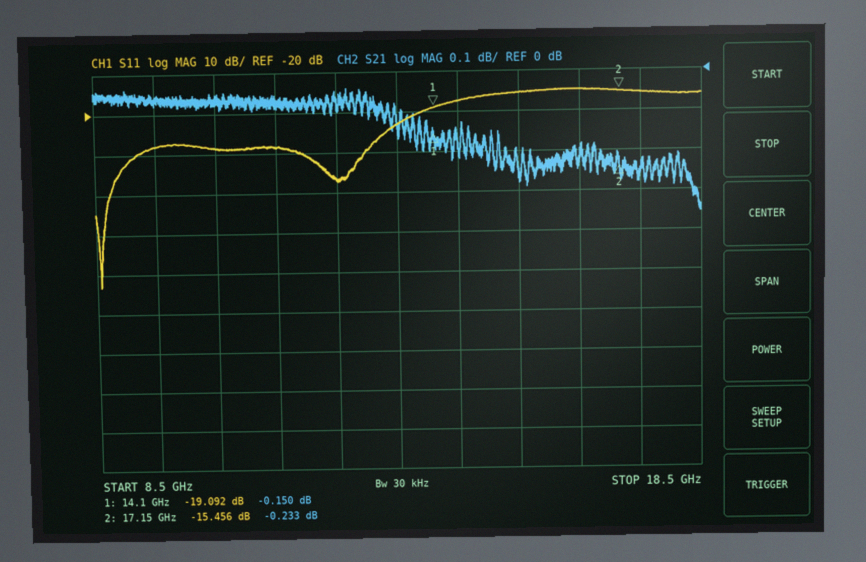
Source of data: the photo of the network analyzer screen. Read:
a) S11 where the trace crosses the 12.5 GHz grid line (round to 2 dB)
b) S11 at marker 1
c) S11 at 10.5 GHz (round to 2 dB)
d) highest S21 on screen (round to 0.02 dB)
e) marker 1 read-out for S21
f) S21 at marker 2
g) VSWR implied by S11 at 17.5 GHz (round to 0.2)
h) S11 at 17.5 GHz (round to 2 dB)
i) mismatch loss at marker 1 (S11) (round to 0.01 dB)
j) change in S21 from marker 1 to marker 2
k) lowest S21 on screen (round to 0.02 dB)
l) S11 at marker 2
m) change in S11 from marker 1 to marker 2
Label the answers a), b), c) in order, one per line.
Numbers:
a) -36 dB
b) -19.092 dB
c) -28 dB
d) -0.04 dB
e) -0.150 dB
f) -0.233 dB
g) 1.4
h) -16 dB
i) 0.05 dB
j) -0.083 dB
k) -0.36 dB
l) -15.456 dB
m) 3.636 dB
